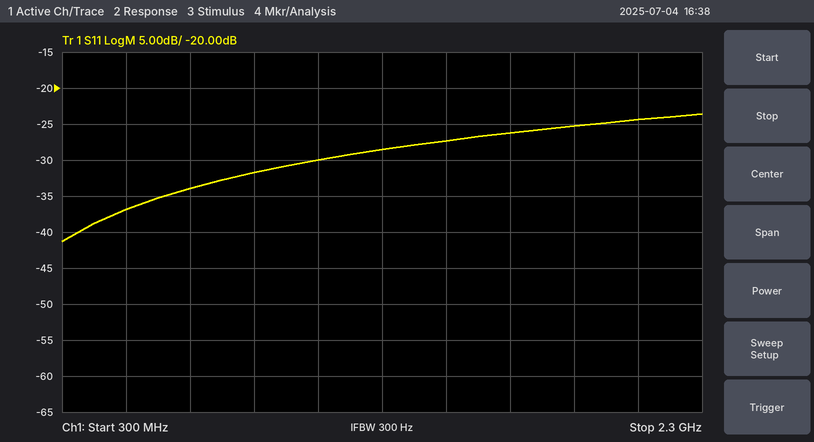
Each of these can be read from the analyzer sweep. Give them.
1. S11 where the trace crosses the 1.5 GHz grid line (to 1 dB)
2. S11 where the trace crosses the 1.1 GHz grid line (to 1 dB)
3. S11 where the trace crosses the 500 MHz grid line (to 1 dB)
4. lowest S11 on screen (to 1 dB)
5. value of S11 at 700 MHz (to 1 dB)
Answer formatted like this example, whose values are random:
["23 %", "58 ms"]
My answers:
["-27 dB", "-30 dB", "-37 dB", "-41 dB", "-34 dB"]
